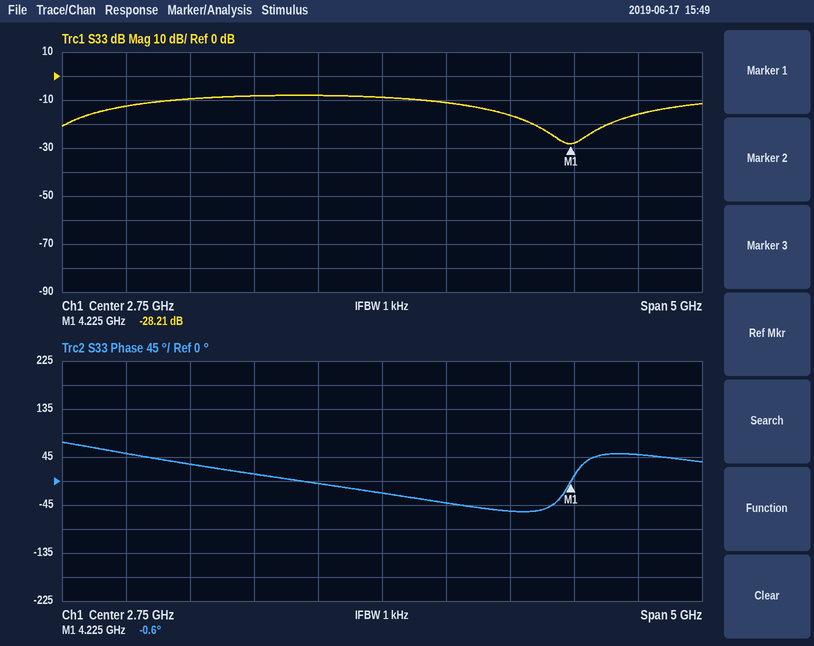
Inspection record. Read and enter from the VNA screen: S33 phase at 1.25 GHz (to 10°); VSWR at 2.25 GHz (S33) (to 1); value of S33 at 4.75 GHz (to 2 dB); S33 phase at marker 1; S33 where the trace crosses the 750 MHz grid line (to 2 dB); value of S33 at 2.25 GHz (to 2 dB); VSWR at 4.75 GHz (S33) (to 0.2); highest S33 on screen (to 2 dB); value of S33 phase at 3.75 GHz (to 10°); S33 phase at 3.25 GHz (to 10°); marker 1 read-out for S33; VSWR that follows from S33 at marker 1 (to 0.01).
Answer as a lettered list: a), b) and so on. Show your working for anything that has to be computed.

a) 30°
b) |Γ| = 10^(-8/20) = 0.3981; VSWR = (1 + 0.3981)/(1 − 0.3981) ≈ 2
c) -16 dB
d) -0.6°
e) -12 dB
f) -8 dB
g) |Γ| = 10^(-16/20) = 0.1585; VSWR = (1 + 0.1585)/(1 − 0.1585) ≈ 1.4
h) -8 dB
i) -60°
j) -40°
k) -28.21 dB
l) (1 + 0.0389)/(1 − 0.0389) ≈ 1.08
